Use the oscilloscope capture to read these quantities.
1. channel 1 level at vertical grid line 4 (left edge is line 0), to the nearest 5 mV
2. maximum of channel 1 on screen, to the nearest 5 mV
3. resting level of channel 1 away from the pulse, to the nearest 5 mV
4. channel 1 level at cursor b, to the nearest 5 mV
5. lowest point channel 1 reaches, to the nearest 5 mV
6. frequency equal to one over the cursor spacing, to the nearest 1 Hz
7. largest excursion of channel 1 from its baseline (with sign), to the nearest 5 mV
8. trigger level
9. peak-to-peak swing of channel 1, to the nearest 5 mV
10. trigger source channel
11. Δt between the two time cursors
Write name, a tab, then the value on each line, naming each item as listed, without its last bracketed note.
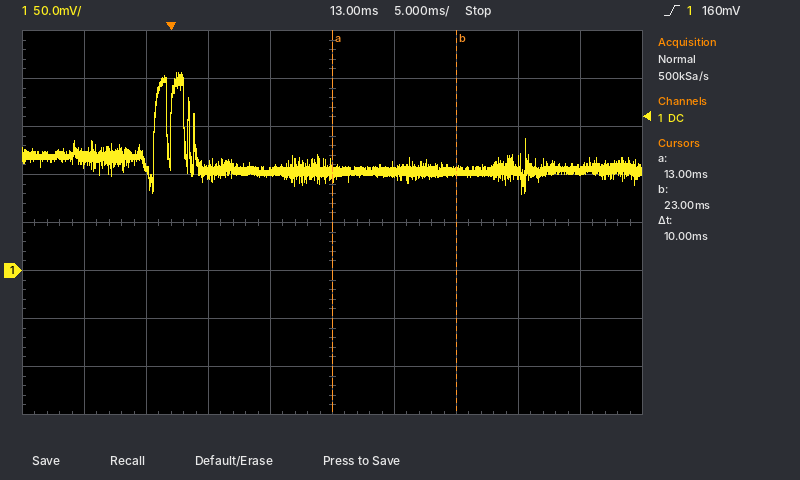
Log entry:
channel 1 level at vertical grid line 4 (left edge is line 0), to the nearest 5 mV	105 mV
maximum of channel 1 on screen, to the nearest 5 mV	205 mV
resting level of channel 1 away from the pulse, to the nearest 5 mV	105 mV
channel 1 level at cursor b, to the nearest 5 mV	105 mV
lowest point channel 1 reaches, to the nearest 5 mV	80 mV
frequency equal to one over the cursor spacing, to the nearest 1 Hz	100 Hz
largest excursion of channel 1 from its baseline (with sign), to the nearest 5 mV	+100 mV
trigger level	160 mV
peak-to-peak swing of channel 1, to the nearest 5 mV	125 mV
trigger source channel	channel 1
Δt between the two time cursors	10 ms
